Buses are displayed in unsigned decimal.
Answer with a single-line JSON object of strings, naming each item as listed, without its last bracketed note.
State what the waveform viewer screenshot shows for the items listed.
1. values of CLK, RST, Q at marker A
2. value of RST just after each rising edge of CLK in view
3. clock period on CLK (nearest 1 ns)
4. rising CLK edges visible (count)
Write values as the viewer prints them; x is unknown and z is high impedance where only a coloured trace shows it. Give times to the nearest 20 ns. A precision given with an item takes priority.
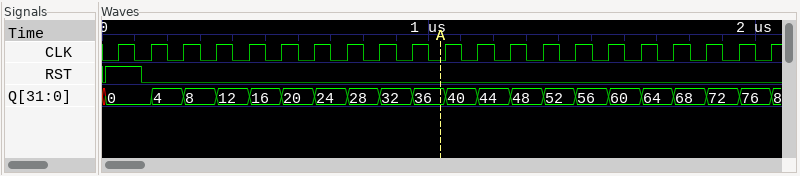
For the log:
{"values of CLK, RST, Q at marker A": "CLK=0, RST=0, Q=36", "value of RST just after each rising edge of CLK in view": "1 0 0 0 0 0 0 0 0 0 0 0 0 0 0 0 0 0 0 0 0", "clock period on CLK": "100 ns", "rising CLK edges visible": "21"}
